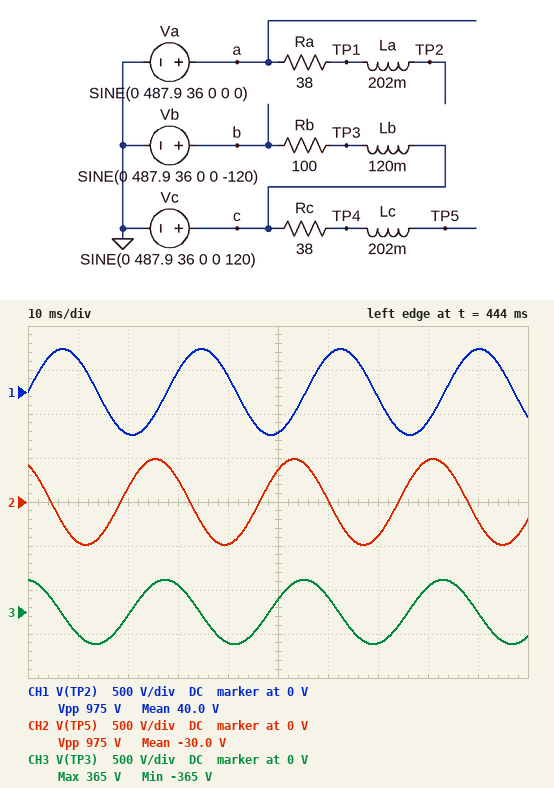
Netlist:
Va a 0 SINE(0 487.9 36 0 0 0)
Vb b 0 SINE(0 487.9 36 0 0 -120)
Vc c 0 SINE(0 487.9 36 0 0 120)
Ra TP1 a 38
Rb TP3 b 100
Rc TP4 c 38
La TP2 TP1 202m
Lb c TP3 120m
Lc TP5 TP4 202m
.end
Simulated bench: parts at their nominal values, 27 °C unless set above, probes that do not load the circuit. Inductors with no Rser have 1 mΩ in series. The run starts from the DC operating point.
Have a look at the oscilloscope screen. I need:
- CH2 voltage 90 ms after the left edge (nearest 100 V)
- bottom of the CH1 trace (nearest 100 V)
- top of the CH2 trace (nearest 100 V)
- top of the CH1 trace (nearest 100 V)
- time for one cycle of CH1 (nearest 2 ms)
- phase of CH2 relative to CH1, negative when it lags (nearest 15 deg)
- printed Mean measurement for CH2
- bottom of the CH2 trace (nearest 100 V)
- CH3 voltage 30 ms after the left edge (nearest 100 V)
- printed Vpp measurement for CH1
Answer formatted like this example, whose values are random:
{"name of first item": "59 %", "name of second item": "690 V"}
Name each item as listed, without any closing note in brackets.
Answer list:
{"CH2 voltage 90 ms after the left edge": "-200 V", "bottom of the CH1 trace": "-500 V", "top of the CH2 trace": "500 V", "top of the CH1 trace": "500 V", "time for one cycle of CH1": "28 ms", "phase of CH2 relative to CH1, negative when it lags": "120 deg", "printed Mean measurement for CH2": "-30.0 V", "bottom of the CH2 trace": "-500 V", "CH3 voltage 30 ms after the left edge": "300 V", "printed Vpp measurement for CH1": "975 V"}
